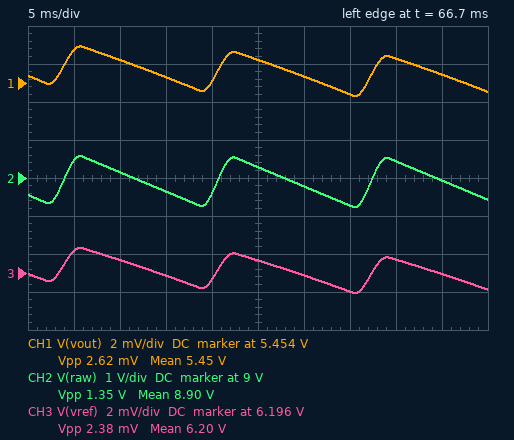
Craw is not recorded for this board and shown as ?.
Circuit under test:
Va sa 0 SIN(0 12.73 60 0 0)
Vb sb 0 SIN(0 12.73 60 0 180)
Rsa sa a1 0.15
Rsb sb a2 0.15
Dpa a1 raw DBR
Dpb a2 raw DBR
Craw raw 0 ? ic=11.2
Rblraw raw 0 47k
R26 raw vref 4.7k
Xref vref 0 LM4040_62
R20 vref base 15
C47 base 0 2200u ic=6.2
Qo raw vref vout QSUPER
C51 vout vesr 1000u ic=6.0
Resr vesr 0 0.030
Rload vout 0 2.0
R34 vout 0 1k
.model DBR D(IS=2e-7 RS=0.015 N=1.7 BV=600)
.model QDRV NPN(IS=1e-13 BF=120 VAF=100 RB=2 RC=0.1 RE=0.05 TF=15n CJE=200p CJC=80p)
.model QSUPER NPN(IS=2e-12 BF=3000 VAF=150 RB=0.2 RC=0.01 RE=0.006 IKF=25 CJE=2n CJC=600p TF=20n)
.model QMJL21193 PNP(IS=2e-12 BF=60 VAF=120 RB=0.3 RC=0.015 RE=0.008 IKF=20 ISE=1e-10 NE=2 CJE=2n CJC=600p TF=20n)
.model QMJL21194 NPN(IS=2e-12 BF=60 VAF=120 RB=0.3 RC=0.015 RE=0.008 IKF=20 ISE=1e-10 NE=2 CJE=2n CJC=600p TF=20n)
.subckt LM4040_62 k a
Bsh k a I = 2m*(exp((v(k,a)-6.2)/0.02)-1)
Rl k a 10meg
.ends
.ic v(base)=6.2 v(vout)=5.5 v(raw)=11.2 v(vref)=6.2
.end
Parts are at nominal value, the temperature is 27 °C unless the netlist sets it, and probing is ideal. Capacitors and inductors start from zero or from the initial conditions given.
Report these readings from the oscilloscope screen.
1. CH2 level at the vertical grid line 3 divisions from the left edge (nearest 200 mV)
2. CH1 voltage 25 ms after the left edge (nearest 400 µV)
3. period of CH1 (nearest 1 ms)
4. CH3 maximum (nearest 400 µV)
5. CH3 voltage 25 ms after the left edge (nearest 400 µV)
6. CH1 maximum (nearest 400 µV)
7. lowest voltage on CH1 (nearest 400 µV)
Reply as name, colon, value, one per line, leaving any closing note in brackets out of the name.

CH2 level at the vertical grid line 3 divisions from the left edge: 8.6 V
CH1 voltage 25 ms after the left edge: 5.4552 V
period of CH1: 17 ms
CH3 maximum: 6.1972 V
CH3 voltage 25 ms after the left edge: 6.1968 V
CH1 maximum: 5.4560 V
lowest voltage on CH1: 5.4532 V
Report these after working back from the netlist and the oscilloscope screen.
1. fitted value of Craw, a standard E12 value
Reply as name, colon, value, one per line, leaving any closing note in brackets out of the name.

fitted value of Craw, a standard E12 value: 27 mF
